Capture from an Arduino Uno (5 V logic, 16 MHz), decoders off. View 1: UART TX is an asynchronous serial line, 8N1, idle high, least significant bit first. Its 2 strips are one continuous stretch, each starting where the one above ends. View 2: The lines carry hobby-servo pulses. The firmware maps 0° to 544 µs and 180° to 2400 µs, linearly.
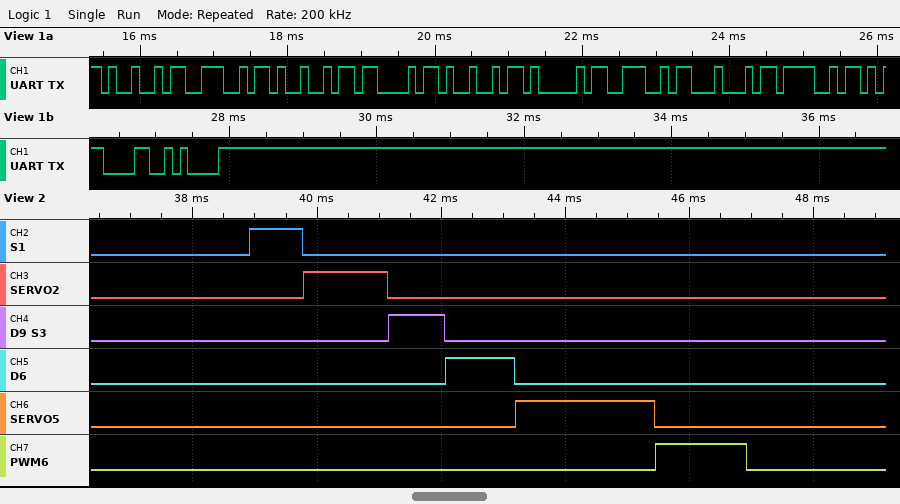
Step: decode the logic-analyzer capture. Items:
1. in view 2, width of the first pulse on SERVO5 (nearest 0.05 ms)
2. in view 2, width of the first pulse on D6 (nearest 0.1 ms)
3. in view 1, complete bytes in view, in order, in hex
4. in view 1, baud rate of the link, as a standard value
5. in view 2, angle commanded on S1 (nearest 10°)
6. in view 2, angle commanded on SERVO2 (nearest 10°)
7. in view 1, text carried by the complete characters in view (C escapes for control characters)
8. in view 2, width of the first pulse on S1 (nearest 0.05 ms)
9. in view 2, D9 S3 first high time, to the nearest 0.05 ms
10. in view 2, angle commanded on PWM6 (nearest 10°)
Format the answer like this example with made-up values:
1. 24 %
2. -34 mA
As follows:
1. 2.25 ms
2. 1.1 ms
3. 49 4E 49 43 49 41 4E 44 4F 0D 0A
4. 9600 baud
5. 30°
6. 80°
7. "INICIANDO\r\n"
8. 0.85 ms
9. 0.90 ms
10. 90°
